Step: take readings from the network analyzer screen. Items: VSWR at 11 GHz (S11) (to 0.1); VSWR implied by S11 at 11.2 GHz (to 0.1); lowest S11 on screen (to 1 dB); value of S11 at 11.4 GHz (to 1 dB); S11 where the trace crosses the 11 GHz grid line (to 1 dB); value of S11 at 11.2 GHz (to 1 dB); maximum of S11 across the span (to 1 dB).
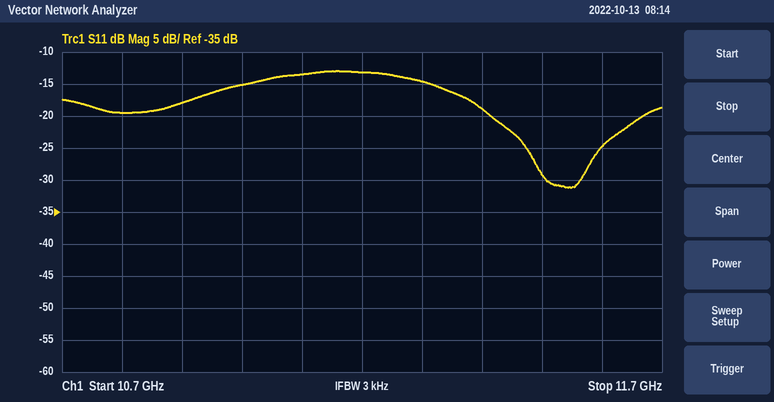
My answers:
1.4
1.6
-31 dB
-19 dB
-15 dB
-13 dB
-13 dB
